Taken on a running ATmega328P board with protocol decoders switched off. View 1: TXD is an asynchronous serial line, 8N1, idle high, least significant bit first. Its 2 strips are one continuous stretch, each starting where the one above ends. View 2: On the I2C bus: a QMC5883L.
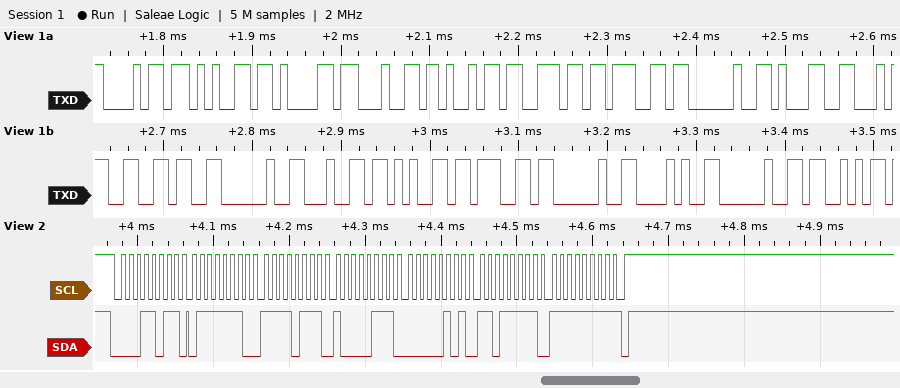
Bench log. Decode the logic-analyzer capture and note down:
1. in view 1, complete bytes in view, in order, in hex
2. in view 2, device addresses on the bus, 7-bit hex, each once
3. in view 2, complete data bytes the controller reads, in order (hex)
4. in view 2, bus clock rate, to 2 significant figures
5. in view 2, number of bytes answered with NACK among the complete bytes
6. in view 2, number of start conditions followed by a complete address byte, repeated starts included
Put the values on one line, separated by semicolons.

68 65 61 64 69 6E 67 20 31 34 36 20 64 65 67 20 28 20 53; 0x0D; 7E F7 87 05 DF FF; 100 kHz; 1; 1
